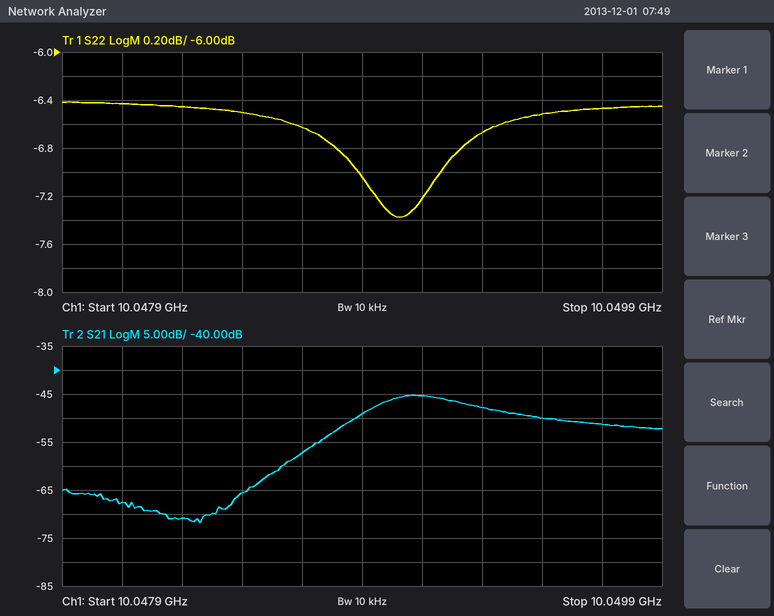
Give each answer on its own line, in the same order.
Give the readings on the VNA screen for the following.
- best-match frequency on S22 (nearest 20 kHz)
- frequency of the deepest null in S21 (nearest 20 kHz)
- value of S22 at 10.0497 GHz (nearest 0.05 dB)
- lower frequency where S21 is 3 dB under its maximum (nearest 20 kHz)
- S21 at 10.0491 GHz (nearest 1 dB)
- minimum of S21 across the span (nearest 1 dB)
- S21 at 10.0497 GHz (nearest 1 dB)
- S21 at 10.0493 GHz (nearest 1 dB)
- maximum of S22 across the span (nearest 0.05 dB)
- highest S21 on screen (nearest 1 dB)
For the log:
10.04902 GHz
10.04836 GHz
-6.45 dB
10.04892 GHz
-45 dB
-72 dB
-51 dB
-48 dB
-6.40 dB
-45 dB
